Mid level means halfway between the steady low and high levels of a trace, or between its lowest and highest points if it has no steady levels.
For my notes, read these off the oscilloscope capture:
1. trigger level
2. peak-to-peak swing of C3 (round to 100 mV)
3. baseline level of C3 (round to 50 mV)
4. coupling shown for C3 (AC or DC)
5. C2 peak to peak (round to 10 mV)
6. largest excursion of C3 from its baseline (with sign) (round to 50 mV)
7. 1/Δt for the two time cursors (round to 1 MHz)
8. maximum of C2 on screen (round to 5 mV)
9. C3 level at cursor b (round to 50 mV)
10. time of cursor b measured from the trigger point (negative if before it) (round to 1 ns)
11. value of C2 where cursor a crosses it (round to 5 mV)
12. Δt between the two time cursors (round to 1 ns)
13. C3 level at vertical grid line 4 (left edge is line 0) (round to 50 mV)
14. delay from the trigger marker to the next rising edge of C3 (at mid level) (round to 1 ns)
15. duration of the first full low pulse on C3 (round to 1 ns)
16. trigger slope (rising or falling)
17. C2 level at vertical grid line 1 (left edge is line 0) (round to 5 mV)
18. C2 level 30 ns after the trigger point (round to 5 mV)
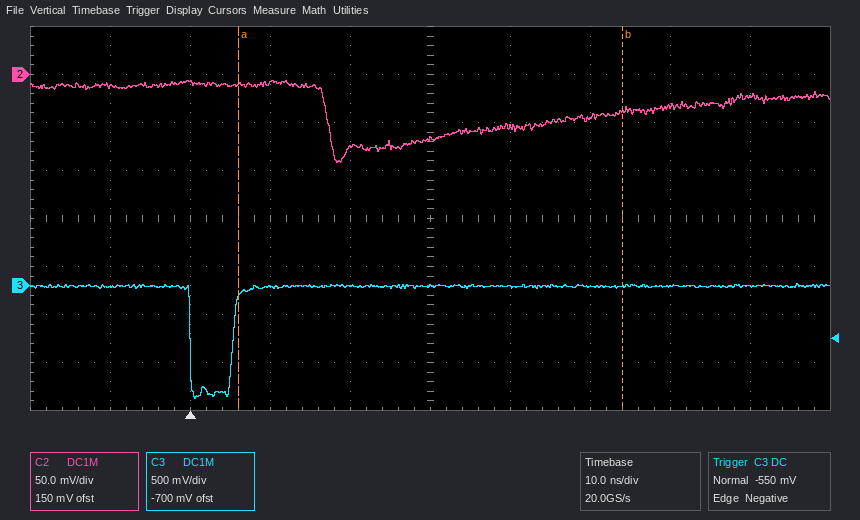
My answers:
-550 mV
1.20 V
0 mV
DC
90 mV
-1.15 V
21 MHz
-5 mV
0 mV
+54 ns
-10 mV
48 ns
0 mV
5 ns
5 ns
falling
-10 mV
-65 mV
